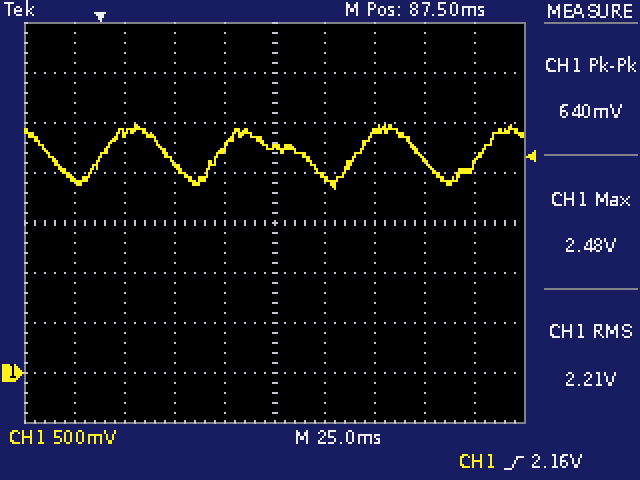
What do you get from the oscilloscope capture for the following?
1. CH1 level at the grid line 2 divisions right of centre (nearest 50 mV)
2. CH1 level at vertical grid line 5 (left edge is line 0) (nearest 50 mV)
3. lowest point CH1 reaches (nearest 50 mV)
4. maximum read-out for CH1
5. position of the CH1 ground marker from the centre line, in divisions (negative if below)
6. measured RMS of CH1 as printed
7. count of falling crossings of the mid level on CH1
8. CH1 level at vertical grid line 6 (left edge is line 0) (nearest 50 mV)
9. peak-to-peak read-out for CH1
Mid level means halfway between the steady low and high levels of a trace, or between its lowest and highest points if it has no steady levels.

2.40 V
2.25 V
1.85 V
2.48 V
-3.0 div
2.21 V
4
1.95 V
640 mV
